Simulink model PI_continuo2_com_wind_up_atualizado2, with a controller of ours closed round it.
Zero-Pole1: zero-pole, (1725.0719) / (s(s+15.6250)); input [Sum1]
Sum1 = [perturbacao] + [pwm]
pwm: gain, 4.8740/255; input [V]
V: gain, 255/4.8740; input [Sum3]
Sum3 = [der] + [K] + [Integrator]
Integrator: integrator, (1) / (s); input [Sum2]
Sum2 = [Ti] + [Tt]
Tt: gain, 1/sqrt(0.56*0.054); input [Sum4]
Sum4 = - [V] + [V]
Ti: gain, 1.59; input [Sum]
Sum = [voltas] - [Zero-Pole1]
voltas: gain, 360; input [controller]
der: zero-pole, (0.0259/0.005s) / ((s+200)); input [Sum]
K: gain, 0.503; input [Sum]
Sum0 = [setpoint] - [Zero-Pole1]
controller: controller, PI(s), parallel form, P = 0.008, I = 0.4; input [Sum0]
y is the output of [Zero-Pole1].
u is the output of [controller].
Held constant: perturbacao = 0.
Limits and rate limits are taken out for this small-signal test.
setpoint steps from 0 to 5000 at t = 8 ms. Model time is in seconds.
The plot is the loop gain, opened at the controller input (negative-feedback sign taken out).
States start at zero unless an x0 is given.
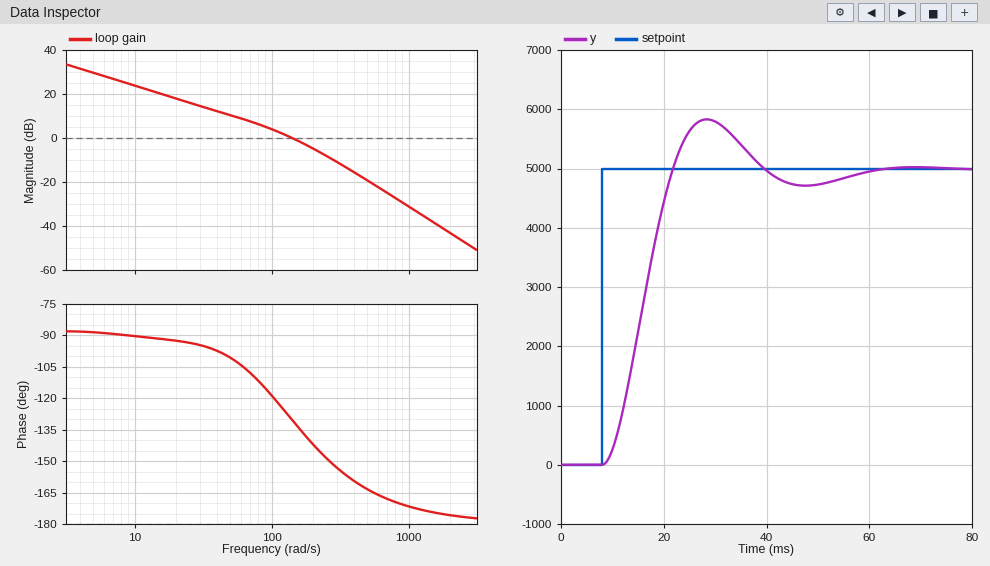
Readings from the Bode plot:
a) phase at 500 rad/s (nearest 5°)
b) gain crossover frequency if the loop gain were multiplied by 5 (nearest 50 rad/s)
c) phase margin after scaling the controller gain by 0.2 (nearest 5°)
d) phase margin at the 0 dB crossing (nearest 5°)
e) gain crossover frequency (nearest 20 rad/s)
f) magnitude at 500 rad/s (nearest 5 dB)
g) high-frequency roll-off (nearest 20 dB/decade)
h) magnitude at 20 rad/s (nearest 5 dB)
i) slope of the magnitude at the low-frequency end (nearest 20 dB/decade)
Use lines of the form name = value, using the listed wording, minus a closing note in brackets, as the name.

phase at 500 rad/s = -165°
gain crossover frequency if the loop gain were multiplied by 5 = 350 rad/s
phase margin after scaling the controller gain by 0.2 = 85°
phase margin at the 0 dB crossing = 50°
gain crossover frequency = 140 rad/s
magnitude at 500 rad/s = -20 dB
high-frequency roll-off = -40 dB/decade
magnitude at 20 rad/s = 20 dB
slope of the magnitude at the low-frequency end = -20 dB/decade
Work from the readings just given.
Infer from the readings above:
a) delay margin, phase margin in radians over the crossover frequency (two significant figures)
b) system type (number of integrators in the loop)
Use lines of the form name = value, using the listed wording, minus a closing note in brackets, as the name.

delay margin, phase margin in radians over the crossover frequency = 0.0062 s
system type = 1
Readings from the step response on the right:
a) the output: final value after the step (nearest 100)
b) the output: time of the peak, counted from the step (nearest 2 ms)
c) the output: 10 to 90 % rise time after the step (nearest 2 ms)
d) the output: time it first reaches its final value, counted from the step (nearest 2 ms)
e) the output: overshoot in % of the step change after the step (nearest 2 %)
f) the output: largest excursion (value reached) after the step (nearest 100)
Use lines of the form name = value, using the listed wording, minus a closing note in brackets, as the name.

the output: final value after the step = 5000
the output: time of the peak, counted from the step = 20 ms
the output: 10 to 90 % rise time after the step = 10 ms
the output: time it first reaches its final value, counted from the step = 14 ms
the output: overshoot in % of the step change after the step = 16 %
the output: largest excursion (value reached) after the step = 5800
